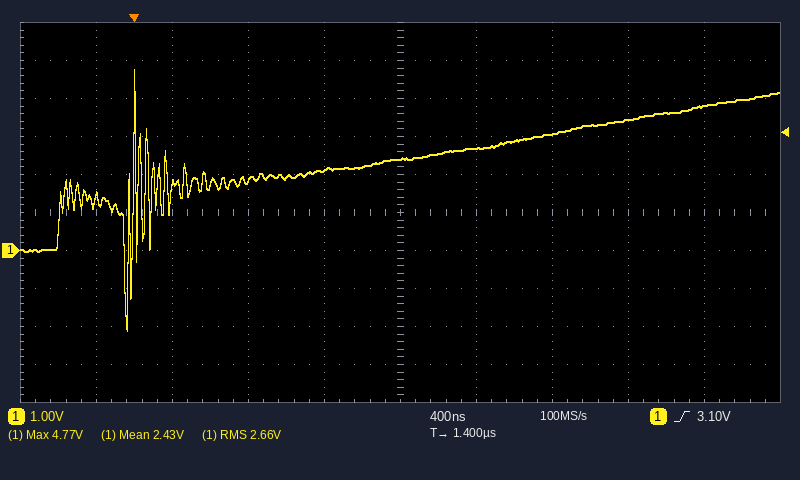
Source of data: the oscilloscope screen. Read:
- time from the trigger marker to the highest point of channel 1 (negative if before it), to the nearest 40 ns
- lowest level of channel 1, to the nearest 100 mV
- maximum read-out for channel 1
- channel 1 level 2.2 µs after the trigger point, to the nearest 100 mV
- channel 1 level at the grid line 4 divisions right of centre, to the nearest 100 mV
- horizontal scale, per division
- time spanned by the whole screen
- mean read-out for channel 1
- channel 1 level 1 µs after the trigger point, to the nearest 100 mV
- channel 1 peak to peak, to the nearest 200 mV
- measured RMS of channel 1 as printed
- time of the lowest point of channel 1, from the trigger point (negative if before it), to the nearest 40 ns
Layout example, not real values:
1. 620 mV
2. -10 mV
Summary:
1. 0 ns
2. -2.1 V
3. 4.77 V
4. 3.1 V
5. 3.8 V
6. 400 ns
7. 4 µs
8. 2.43 V
9. 2.1 V
10. 6.8 V
11. 2.66 V
12. -40 ns
